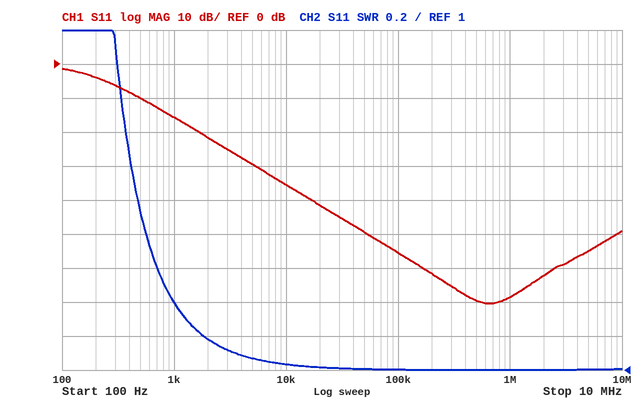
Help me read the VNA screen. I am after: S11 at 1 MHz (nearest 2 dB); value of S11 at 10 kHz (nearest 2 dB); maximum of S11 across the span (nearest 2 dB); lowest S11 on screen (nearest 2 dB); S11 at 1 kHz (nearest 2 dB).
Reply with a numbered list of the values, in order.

1. -68 dB
2. -36 dB
3. -2 dB
4. -70 dB
5. -16 dB
